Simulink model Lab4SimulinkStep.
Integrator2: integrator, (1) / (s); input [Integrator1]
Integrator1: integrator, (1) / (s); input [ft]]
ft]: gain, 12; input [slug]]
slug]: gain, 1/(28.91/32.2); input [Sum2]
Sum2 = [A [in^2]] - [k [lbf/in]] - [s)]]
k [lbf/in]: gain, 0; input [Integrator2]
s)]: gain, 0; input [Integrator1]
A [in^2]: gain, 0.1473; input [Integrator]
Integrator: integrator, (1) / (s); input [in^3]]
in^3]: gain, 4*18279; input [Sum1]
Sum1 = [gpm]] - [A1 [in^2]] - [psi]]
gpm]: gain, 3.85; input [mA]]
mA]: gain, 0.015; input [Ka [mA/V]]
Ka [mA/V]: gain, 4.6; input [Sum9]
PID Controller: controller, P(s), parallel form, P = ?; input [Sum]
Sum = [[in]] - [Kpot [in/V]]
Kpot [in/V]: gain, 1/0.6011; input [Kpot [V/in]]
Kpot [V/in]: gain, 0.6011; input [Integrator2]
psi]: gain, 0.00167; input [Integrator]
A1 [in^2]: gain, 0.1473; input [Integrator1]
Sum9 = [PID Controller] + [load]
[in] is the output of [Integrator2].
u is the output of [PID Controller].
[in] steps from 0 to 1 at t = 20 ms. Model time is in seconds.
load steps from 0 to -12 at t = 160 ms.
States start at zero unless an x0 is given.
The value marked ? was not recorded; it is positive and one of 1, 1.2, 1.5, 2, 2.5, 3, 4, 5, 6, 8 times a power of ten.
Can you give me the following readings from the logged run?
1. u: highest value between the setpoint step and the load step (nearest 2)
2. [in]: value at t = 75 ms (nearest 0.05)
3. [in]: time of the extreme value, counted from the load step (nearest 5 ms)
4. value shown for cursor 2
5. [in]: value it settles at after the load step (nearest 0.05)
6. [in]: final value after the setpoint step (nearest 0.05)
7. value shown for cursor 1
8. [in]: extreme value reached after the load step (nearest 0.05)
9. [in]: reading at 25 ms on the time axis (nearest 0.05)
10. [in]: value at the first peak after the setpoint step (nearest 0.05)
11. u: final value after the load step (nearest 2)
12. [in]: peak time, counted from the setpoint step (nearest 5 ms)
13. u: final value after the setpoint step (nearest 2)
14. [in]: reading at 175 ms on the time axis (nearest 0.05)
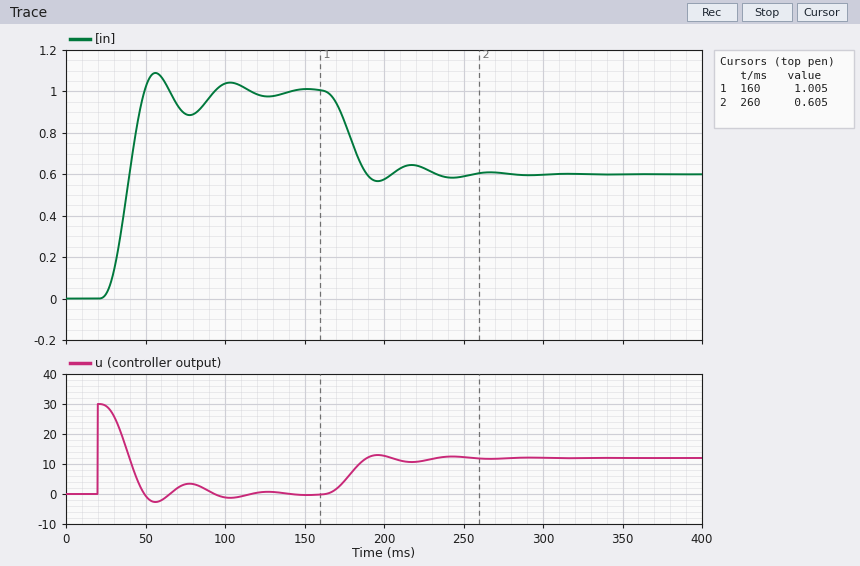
30
0.90
35 ms
0.605
0.60
1.00
1.005
0.55
0.00
1.10
12
35 ms
0
0.85
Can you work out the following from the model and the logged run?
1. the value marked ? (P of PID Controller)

30
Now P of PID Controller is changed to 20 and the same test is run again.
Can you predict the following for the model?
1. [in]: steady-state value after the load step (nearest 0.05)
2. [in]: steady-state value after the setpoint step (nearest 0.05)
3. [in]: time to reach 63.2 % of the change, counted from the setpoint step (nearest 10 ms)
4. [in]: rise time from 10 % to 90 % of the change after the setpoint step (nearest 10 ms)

0.40
1.00
30 ms
50 ms
